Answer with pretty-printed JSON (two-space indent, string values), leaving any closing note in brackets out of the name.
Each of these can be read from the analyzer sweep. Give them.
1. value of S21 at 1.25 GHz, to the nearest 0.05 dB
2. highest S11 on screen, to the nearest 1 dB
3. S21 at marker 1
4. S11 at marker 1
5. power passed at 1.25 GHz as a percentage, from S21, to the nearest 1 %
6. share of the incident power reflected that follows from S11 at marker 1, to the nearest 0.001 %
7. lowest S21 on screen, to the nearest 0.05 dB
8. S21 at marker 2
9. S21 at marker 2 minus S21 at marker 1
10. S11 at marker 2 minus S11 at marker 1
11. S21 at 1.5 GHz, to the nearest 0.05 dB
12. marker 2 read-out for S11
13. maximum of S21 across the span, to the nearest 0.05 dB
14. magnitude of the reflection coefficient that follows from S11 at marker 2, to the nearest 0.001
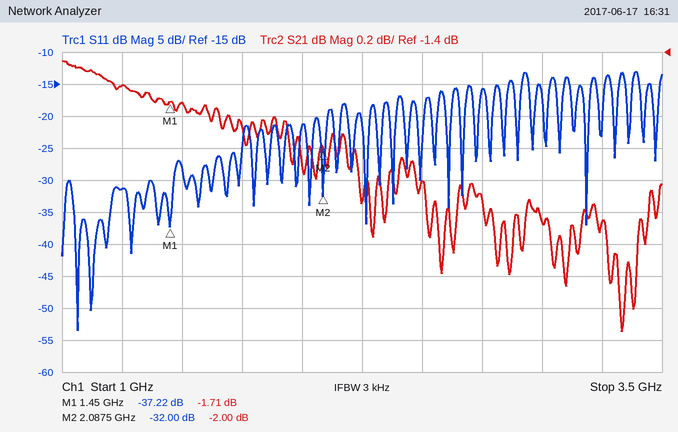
{
  "value of S21 at 1.25 GHz, to the nearest 0.05 dB": "-1.60 dB",
  "highest S11 on screen, to the nearest 1 dB": "-13 dB",
  "S21 at marker 1": "-1.71 dB",
  "S11 at marker 1": "-37.22 dB",
  "power passed at 1.25 GHz as a percentage, from S21, to the nearest 1 %": "69 %",
  "share of the incident power reflected that follows from S11 at marker 1, to the nearest 0.001 %": "0.019 %",
  "lowest S21 on screen, to the nearest 0.05 dB": "-3.15 dB",
  "S21 at marker 2": "-2.00 dB",
  "S21 at marker 2 minus S21 at marker 1": "-0.29 dB",
  "S11 at marker 2 minus S11 at marker 1": "5.22 dB",
  "S21 at 1.5 GHz, to the nearest 0.05 dB": "-1.70 dB",
  "marker 2 read-out for S11": "-32.00 dB",
  "maximum of S21 across the span, to the nearest 0.05 dB": "-1.45 dB",
  "magnitude of the reflection coefficient that follows from S11 at marker 2, to the nearest 0.001": "0.025"
}
